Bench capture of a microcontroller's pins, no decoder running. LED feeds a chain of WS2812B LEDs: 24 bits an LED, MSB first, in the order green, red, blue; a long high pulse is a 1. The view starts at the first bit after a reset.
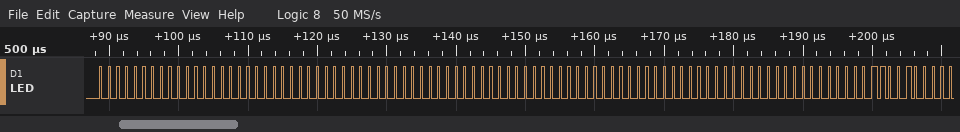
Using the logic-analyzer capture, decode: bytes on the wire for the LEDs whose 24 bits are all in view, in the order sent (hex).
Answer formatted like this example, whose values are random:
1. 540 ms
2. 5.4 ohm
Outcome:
1. 00 00 00 00 00 00 00 00 00 00 00 64
